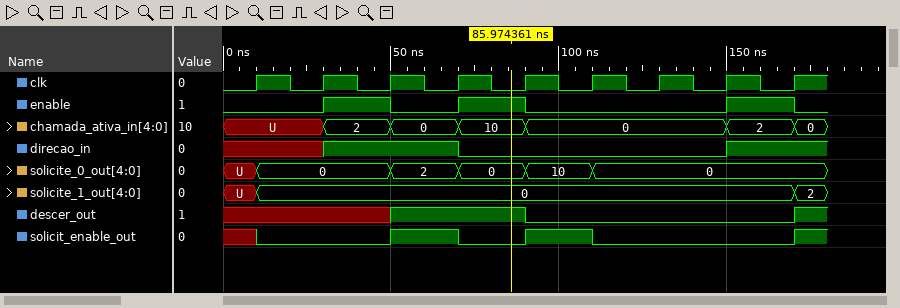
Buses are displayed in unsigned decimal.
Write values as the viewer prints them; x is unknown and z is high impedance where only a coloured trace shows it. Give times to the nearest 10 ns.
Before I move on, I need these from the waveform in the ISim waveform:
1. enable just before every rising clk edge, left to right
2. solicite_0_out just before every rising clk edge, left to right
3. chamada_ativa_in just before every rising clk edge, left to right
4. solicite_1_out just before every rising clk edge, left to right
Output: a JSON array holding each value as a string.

["0 0 1 0 1 0 0 0 1", "U, 0, 0, 2, 0, 10, 0, 0, 0", "U, U, 2, 0, 10, 0, 0, 0, 2", "U, 0, 0, 0, 0, 0, 0, 0, 0"]
